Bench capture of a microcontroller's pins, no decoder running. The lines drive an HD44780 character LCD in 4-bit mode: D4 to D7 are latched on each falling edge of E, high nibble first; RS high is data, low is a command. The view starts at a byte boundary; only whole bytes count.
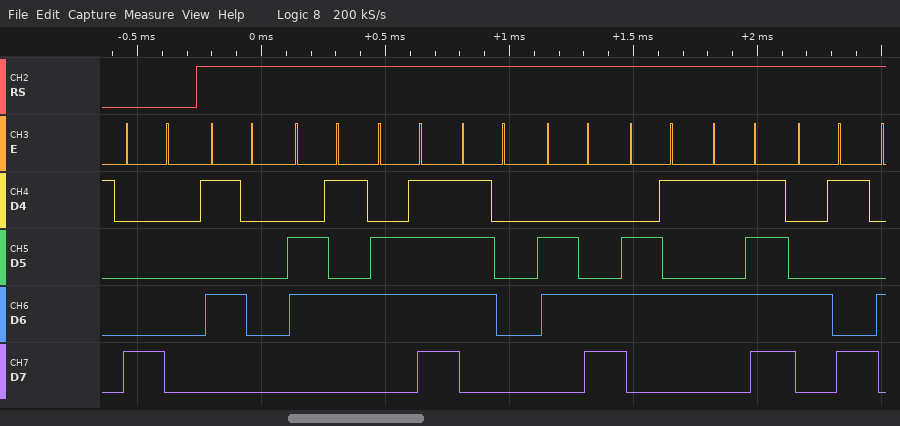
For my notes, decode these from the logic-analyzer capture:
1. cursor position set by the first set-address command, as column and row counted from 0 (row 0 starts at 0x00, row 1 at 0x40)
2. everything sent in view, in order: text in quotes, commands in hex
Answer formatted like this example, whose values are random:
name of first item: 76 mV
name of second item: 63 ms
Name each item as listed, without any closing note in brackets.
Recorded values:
cursor position set by the first set-address command, as column and row counted from 0: column 0, row 0
everything sent in view, in order: text in quotes, commands in hex: 0x80 "People_I"
